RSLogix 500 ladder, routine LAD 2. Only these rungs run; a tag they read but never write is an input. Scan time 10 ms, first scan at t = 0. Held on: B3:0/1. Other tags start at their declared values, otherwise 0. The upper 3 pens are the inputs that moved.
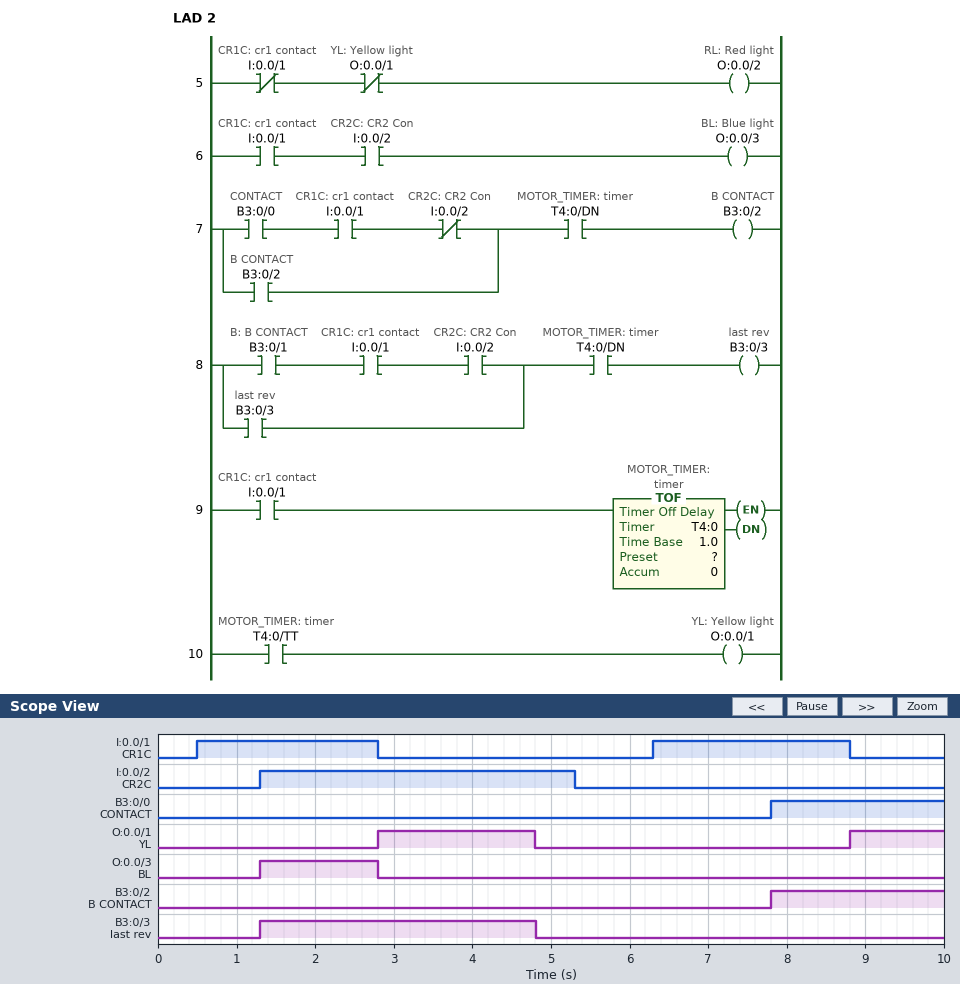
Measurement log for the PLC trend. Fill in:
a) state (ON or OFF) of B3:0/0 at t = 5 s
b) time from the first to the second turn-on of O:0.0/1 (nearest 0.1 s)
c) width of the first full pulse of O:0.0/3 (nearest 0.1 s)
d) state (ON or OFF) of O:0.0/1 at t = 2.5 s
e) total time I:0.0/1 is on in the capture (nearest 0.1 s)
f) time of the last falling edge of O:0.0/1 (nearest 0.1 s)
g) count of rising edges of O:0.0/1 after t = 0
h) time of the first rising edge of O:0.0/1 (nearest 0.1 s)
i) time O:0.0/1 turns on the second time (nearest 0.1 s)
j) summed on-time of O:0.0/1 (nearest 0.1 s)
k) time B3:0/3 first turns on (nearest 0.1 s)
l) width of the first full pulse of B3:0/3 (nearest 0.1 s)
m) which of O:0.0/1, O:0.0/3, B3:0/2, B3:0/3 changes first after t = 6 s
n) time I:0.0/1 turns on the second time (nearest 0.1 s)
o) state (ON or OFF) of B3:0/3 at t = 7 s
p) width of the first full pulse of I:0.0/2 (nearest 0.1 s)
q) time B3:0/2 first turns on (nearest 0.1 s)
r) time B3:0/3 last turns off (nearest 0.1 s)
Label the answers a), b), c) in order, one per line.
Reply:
a) OFF
b) 6.0 s
c) 1.5 s
d) OFF
e) 4.8 s
f) 4.8 s
g) 2
h) 2.8 s
i) 8.8 s
j) 3.2 s
k) 1.3 s
l) 3.5 s
m) B3:0/2
n) 6.3 s
o) OFF
p) 4.0 s
q) 7.8 s
r) 4.8 s
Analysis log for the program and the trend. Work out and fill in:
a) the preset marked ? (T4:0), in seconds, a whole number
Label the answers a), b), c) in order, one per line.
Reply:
a) 2 s
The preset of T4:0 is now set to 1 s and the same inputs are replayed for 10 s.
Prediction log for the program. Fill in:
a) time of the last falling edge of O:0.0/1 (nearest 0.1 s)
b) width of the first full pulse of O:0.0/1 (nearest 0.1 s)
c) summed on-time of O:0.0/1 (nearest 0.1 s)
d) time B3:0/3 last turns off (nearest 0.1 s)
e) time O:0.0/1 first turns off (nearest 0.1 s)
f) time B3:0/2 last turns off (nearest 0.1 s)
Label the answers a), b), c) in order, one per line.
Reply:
a) 9.8 s
b) 1.0 s
c) 2.0 s
d) 3.8 s
e) 3.8 s
f) 9.8 s
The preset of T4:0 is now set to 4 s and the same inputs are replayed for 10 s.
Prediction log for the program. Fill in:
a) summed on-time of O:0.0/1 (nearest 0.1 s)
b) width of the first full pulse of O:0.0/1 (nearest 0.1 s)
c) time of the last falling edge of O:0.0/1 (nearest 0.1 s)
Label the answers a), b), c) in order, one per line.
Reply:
a) 4.7 s
b) 3.5 s
c) 6.3 s
